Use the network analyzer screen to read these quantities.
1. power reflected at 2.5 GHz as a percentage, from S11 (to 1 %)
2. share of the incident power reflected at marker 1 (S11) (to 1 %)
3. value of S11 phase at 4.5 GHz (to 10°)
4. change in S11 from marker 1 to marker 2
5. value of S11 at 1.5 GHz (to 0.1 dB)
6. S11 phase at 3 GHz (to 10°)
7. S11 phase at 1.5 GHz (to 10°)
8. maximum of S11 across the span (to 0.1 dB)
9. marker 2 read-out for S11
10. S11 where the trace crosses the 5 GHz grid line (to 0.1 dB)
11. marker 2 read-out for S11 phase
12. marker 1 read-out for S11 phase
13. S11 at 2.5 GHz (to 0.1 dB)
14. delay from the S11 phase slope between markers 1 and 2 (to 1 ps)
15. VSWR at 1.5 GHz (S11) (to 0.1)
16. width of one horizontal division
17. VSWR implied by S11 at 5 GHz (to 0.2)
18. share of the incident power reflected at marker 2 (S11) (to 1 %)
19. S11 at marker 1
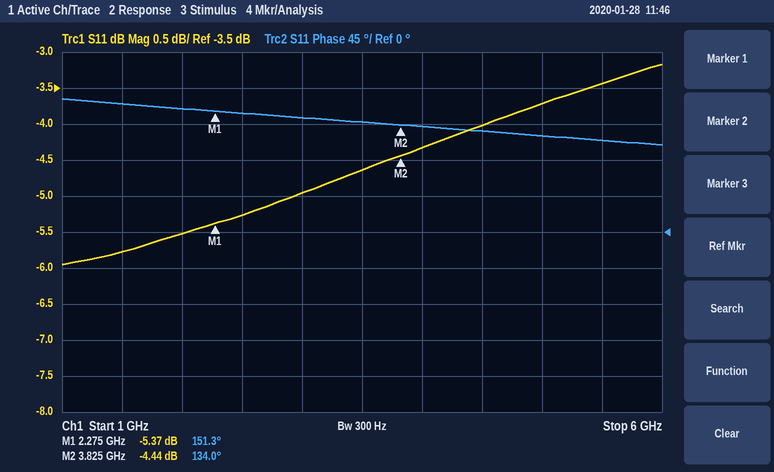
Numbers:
30 %
29 %
130°
0.93 dB
-5.8 dB
140°
160°
-3.2 dB
-4.44 dB
-3.7 dB
134.0°
151.3°
-5.3 dB
31 ps
3.1
500 MHz
4.8
36 %
-5.37 dB
